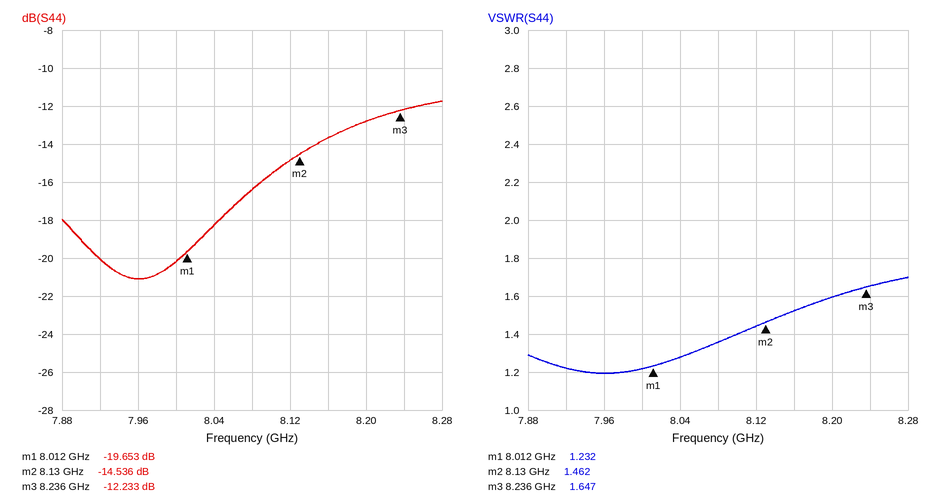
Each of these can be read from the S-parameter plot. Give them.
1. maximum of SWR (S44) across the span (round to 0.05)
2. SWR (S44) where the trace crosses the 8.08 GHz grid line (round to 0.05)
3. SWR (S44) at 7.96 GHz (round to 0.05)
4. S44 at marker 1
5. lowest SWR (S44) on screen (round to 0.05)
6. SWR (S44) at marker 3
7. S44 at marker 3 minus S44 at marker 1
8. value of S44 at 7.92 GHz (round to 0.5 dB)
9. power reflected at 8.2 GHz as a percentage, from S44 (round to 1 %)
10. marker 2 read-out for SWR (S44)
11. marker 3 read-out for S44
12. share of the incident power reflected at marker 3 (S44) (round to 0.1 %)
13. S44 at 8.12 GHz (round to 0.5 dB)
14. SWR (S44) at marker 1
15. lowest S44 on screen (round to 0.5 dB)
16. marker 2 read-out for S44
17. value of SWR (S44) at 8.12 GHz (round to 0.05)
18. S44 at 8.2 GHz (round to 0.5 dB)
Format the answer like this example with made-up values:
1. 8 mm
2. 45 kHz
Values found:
1. 1.70
2. 1.35
3. 1.20
4. -19.653 dB
5. 1.20
6. 1.647
7. 7.420 dB
8. -20.0 dB
9. 5 %
10. 1.462
11. -12.233 dB
12. 6.0 %
13. -15.0 dB
14. 1.232
15. -21.0 dB
16. -14.536 dB
17. 1.45
18. -13.0 dB
